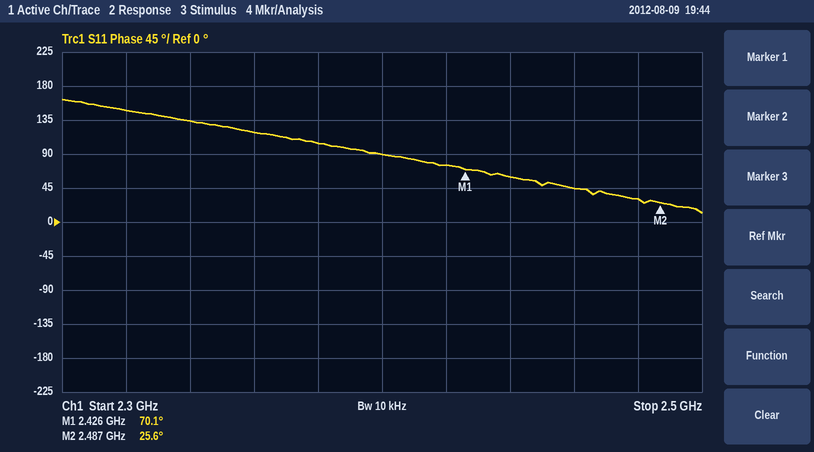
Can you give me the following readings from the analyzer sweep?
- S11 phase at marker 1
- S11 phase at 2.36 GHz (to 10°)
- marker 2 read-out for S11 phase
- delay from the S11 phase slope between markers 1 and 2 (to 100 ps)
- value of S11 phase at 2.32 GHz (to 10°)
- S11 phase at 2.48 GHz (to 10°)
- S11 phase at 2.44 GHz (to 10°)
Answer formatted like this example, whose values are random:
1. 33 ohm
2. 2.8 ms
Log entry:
1. 70.1°
2. 120°
3. 25.6°
4. 2.0 ns
5. 150°
6. 30°
7. 60°
